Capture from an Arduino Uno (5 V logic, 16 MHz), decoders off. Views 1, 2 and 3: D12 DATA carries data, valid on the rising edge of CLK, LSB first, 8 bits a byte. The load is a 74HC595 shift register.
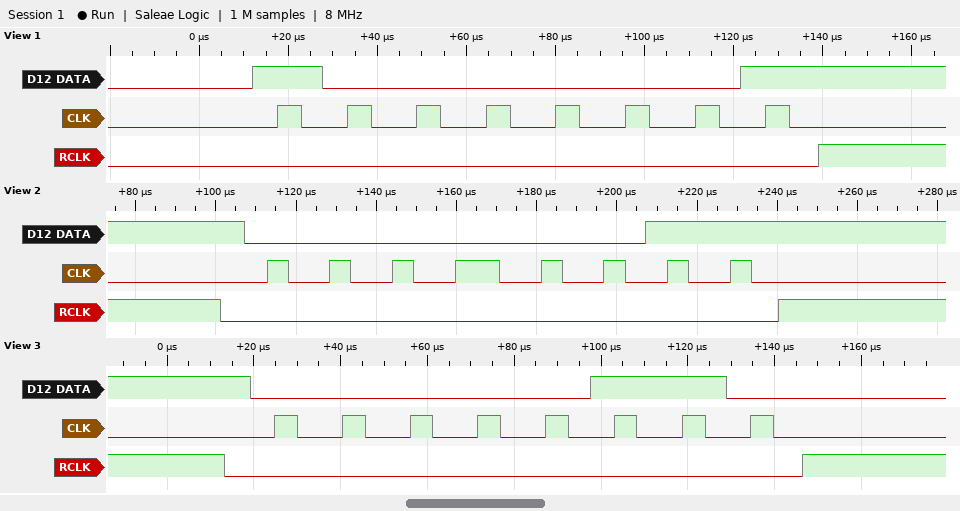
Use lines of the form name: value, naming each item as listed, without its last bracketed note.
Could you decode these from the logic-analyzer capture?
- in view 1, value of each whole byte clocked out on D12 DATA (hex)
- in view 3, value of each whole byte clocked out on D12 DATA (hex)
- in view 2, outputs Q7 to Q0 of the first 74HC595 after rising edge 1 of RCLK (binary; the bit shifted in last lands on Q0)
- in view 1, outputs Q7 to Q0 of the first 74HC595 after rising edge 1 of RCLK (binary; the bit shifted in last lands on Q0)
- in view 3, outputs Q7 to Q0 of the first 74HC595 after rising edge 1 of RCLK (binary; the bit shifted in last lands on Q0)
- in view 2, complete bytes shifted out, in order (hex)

in view 1, value of each whole byte clocked out on D12 DATA: 81
in view 3, value of each whole byte clocked out on D12 DATA: 60
in view 2, outputs Q7 to Q0 of the first 74HC595 after rising edge 1 of RCLK: 00000011
in view 1, outputs Q7 to Q0 of the first 74HC595 after rising edge 1 of RCLK: 10000001
in view 3, outputs Q7 to Q0 of the first 74HC595 after rising edge 1 of RCLK: 00000110
in view 2, complete bytes shifted out, in order: C0
